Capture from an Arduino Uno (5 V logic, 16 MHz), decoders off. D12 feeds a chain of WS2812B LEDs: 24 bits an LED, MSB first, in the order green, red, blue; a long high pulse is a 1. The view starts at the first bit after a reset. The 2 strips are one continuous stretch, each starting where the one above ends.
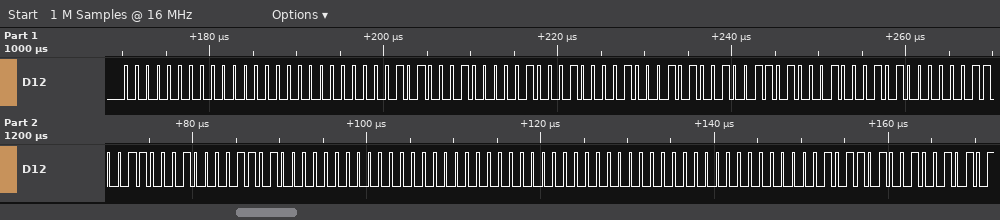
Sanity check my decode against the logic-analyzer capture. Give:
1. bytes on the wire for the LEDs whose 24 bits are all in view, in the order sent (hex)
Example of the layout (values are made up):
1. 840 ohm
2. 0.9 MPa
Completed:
1. 00 00 00 51 04 42 29 34 45 03 31 0D 00 00 00 00 00 00
